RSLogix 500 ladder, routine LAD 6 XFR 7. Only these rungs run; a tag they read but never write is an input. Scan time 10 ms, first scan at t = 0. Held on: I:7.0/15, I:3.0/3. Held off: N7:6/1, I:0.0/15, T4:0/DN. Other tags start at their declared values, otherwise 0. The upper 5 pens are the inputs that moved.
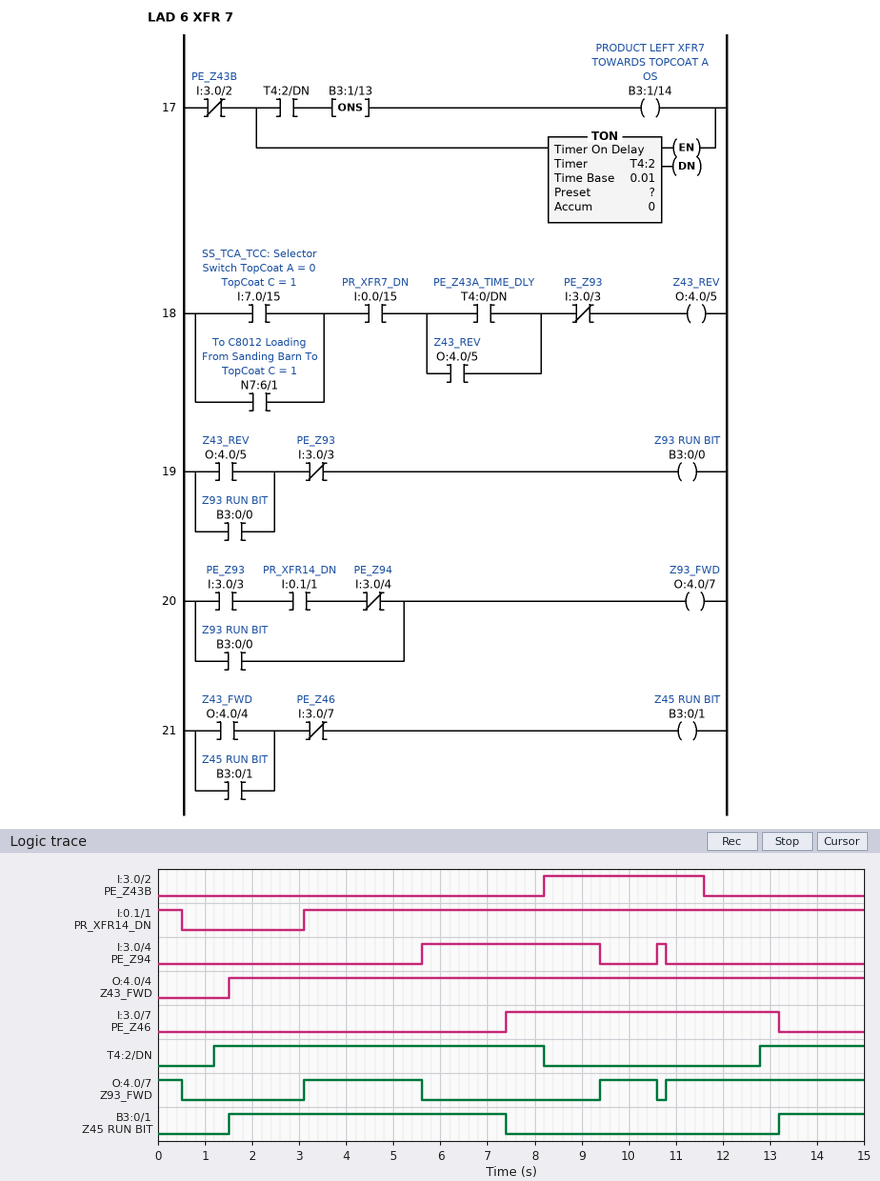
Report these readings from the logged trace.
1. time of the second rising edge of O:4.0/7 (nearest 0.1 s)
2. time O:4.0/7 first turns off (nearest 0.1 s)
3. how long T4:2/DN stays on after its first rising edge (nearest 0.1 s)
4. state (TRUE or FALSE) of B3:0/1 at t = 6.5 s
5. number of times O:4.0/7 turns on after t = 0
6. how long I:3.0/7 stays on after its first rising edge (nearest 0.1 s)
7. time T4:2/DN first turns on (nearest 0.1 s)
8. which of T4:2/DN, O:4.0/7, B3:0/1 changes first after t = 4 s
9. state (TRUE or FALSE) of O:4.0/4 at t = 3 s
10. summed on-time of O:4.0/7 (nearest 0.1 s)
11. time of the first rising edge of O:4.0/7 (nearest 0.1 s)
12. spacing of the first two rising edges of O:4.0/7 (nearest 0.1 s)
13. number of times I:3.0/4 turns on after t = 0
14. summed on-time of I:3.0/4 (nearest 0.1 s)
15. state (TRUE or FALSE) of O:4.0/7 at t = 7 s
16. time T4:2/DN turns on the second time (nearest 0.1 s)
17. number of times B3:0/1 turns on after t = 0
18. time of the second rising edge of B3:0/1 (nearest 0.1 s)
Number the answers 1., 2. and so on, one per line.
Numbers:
1. 9.4 s
2. 0.5 s
3. 7.0 s
4. TRUE
5. 3
6. 5.8 s
7. 1.2 s
8. O:4.0/7
9. TRUE
10. 8.4 s
11. 3.1 s
12. 6.3 s
13. 2
14. 4.0 s
15. FALSE
16. 12.8 s
17. 2
18. 13.2 s
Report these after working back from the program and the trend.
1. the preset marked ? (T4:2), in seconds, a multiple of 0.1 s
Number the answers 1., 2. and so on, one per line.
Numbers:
1. 1.2 s
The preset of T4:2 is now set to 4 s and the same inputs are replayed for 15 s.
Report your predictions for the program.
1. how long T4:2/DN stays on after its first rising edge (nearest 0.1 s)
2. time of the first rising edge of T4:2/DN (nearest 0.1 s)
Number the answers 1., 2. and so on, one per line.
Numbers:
1. 4.2 s
2. 4.0 s
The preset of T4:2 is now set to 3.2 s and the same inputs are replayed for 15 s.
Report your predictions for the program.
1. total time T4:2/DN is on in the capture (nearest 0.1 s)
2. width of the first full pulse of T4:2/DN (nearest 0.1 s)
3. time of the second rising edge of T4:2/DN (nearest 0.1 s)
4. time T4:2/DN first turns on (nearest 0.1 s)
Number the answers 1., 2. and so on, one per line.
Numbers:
1. 5.2 s
2. 5.0 s
3. 14.8 s
4. 3.2 s
